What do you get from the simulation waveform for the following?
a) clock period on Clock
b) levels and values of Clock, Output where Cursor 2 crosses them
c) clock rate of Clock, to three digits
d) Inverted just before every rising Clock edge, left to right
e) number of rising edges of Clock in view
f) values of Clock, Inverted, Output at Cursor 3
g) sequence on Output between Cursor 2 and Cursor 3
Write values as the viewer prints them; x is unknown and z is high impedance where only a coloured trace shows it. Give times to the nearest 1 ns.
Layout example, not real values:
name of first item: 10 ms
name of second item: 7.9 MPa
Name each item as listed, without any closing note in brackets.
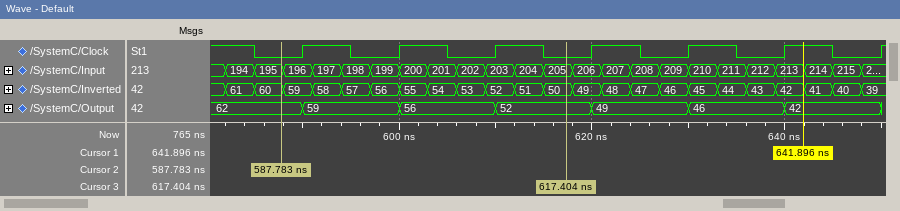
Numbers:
clock period on Clock: 10 ns
levels and values of Clock, Output where Cursor 2 crosses them: Clock=0, Output=62
clock rate of Clock, to three digits: 100 MHz
Inverted just before every rising Clock edge, left to right: 59, 56, 52, 49, 46, 42, 39
number of rising edges of Clock in view: 7
values of Clock, Inverted, Output at Cursor 3: Clock=0, Inverted=50, Output=52
sequence on Output between Cursor 2 and Cursor 3: 62, 59, 56, 52
